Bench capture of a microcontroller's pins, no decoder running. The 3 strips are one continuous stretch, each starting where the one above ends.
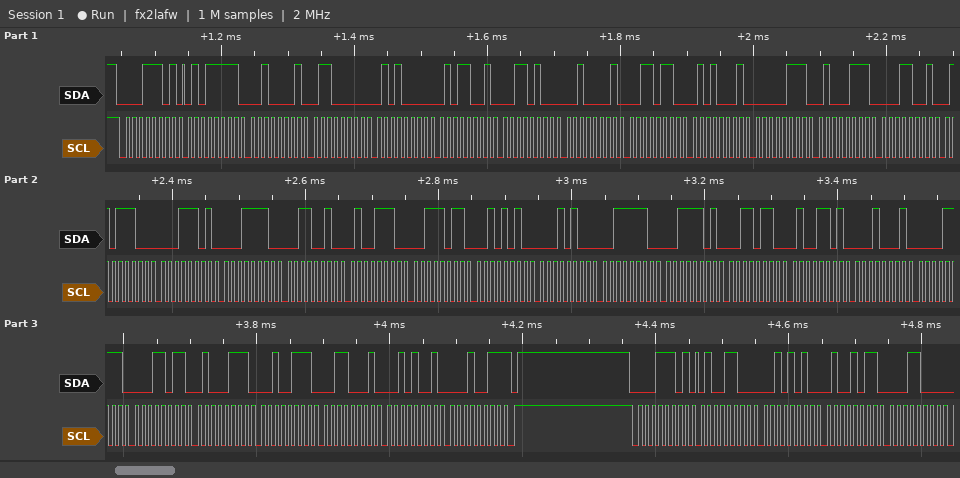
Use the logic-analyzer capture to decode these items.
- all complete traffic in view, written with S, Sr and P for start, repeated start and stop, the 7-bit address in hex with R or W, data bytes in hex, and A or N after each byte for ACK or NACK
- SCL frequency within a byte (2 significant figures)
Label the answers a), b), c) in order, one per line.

a) S 0ER A 5F A 21 A 60 A 50 A 59 A 34 A 21 A 36 A 51 A 07 A 47 A 19 A 5C A 1D A 1E A 32 A 4E A 3B A 2A A 14 A 3E A 3D A 36 A 4D A 11 A 0F A 1B A 47 A 27 A 31 A 29 A 13 N P S 0ER A 4C A 2A A 4B A 18 A
b) 100 kHz
